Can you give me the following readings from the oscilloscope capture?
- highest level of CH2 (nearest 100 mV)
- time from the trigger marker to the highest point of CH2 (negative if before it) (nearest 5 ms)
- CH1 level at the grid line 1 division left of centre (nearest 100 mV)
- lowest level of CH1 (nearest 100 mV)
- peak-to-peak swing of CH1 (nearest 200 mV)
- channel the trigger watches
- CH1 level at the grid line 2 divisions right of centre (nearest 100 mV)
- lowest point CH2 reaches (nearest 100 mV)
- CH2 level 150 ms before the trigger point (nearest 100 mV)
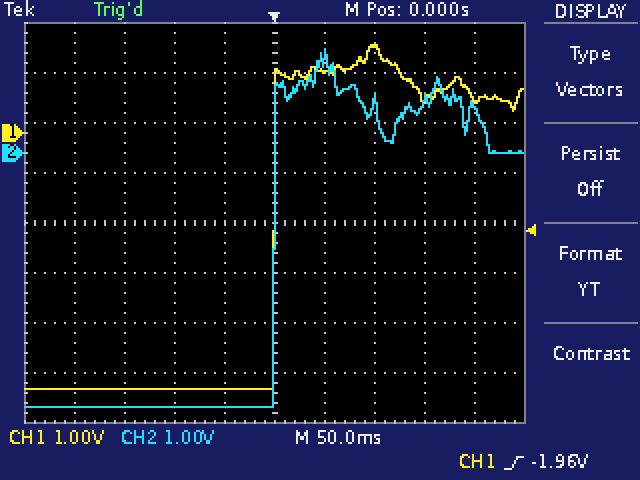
2.1 V
+50 ms
-5.1 V
-5.1 V
6.8 V
CH1
1.7 V
-5.1 V
-5.1 V
